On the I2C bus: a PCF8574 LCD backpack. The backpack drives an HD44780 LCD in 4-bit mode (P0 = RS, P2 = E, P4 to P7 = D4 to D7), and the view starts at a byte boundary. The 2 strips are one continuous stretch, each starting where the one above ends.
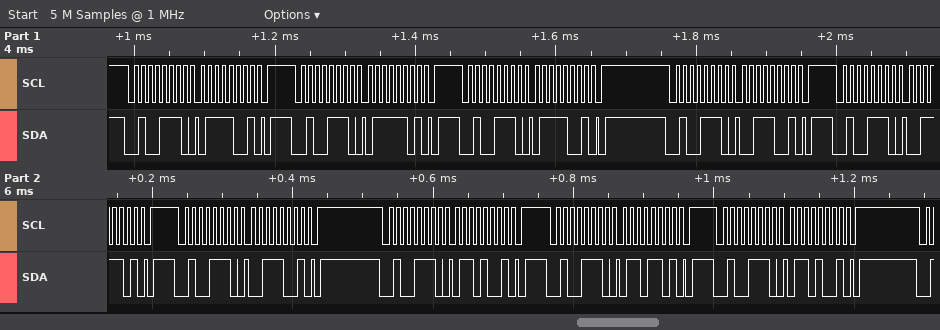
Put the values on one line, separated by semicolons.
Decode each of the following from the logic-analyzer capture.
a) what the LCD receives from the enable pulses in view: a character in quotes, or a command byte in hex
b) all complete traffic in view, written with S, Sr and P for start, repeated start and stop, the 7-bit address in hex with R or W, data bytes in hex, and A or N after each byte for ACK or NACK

's'; S 27W A 79 A P S 27W A 7D A P S 27W A 79 A P S 27W A 39 A P S 27W A 3D A P S 27W A 39 A P S 27W A 69 A P S 27W A 6D A P S 27W A 69 A P
